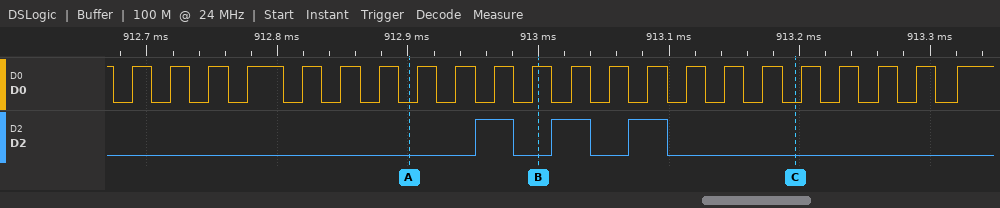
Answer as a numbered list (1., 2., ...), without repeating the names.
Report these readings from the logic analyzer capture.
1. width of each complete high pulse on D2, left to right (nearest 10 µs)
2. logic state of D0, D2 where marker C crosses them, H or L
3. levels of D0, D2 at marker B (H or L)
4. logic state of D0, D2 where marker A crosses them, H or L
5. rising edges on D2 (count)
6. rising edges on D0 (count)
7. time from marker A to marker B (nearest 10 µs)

1. 30 µs, 30 µs, 30 µs
2. D0=L, D2=L
3. D0=H, D2=L
4. D0=L, D2=L
5. 3
6. 22
7. 100 µs
